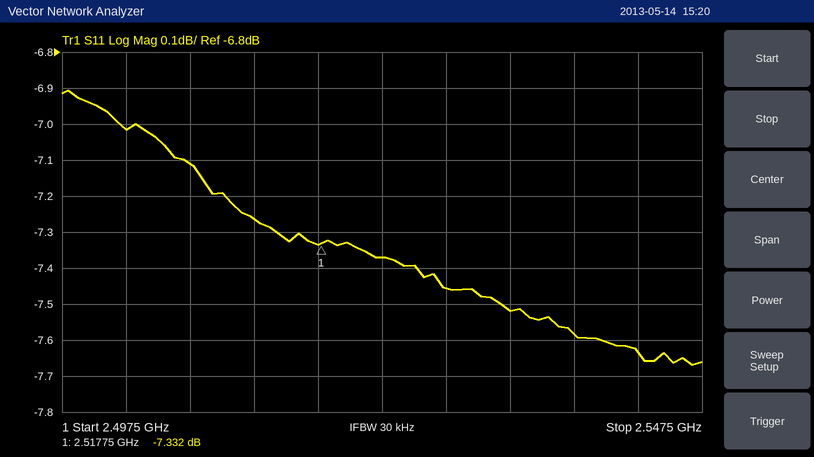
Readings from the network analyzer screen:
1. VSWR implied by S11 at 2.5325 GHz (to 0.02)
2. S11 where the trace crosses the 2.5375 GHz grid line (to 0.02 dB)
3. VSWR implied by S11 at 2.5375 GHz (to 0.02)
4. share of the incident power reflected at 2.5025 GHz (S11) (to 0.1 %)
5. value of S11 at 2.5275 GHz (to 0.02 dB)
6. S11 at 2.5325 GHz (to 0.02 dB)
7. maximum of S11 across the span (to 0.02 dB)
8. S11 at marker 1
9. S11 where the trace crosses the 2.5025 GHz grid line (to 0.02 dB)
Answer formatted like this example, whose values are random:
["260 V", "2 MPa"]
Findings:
["2.46", "-7.58 dB", "2.44", "19.9 %", "-7.46 dB", "-7.52 dB", "-6.90 dB", "-7.332 dB", "-7.02 dB"]
